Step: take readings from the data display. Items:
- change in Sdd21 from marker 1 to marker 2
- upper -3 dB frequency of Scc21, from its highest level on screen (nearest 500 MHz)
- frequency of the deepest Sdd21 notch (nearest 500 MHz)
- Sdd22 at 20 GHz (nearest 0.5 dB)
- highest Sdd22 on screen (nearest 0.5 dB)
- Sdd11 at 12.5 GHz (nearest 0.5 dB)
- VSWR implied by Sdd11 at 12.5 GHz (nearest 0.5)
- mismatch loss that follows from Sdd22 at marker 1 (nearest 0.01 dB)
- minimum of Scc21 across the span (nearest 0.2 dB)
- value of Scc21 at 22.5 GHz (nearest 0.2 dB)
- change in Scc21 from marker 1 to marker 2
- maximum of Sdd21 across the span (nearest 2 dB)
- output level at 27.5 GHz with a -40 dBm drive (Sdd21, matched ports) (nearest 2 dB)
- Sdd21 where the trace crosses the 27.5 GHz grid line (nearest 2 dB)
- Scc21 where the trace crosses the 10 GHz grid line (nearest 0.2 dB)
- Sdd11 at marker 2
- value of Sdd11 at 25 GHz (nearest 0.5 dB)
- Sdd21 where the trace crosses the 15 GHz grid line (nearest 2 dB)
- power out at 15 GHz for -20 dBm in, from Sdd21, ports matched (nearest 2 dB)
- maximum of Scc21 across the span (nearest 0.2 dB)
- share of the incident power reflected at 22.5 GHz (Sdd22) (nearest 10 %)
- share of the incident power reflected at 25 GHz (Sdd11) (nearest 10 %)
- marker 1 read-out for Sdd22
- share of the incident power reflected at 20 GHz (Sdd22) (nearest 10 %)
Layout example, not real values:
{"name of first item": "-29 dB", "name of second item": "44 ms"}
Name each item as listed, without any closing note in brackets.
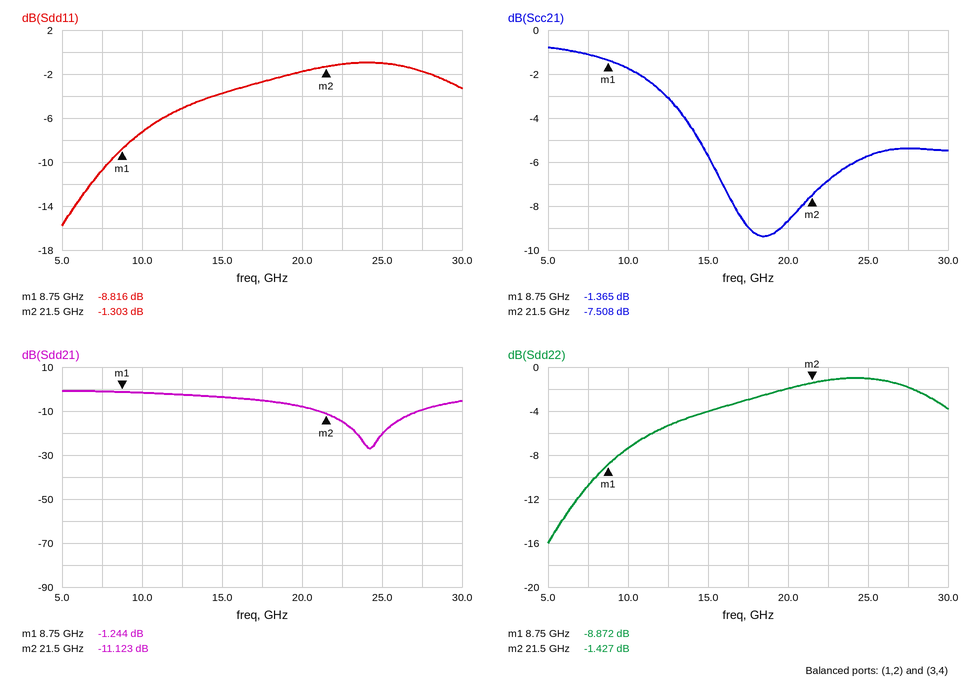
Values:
{"change in Sdd21 from marker 1 to marker 2": "-9.879 dB", "upper -3 dB frequency of Scc21, from its highest level on screen": "13.5 GHz", "frequency of the deepest Sdd21 notch": "24.0 GHz", "Sdd22 at 20 GHz": "-2.0 dB", "highest Sdd22 on screen": "-1.0 dB", "Sdd11 at 12.5 GHz": "-5.0 dB", "VSWR implied by Sdd11 at 12.5 GHz": "3.5", "mismatch loss that follows from Sdd22 at marker 1": "0.60 dB", "minimum of Scc21 across the span": "-9.4 dB", "value of Scc21 at 22.5 GHz": "-6.8 dB", "change in Scc21 from marker 1 to marker 2": "-6.143 dB", "maximum of Sdd21 across the span": "0 dB", "output level at 27.5 GHz with a -40 dBm drive (Sdd21, matched ports)": "-50 dBm", "Sdd21 where the trace crosses the 27.5 GHz grid line": "-10 dB", "Scc21 where the trace crosses the 10 GHz grid line": "-1.8 dB", "Sdd11 at marker 2": "-1.303 dB", "value of Sdd11 at 25 GHz": "-1.0 dB", "Sdd21 where the trace crosses the 15 GHz grid line": "-4 dB", "power out at 15 GHz for -20 dBm in, from Sdd21, ports matched": "-24 dBm", "maximum of Scc21 across the span": "-0.8 dB", "share of the incident power reflected at 22.5 GHz (Sdd22)": "80 %", "share of the incident power reflected at 25 GHz (Sdd11)": "80 %", "marker 1 read-out for Sdd22": "-8.872 dB", "share of the incident power reflected at 20 GHz (Sdd22)": "60 %"}
